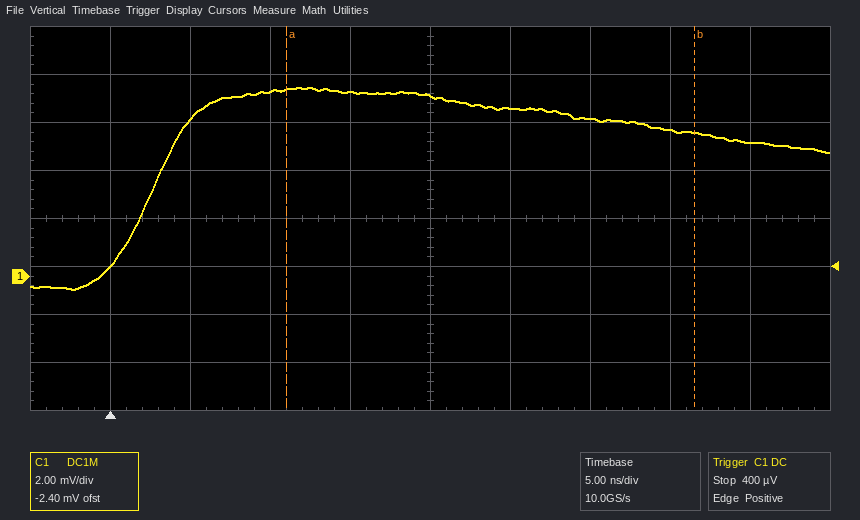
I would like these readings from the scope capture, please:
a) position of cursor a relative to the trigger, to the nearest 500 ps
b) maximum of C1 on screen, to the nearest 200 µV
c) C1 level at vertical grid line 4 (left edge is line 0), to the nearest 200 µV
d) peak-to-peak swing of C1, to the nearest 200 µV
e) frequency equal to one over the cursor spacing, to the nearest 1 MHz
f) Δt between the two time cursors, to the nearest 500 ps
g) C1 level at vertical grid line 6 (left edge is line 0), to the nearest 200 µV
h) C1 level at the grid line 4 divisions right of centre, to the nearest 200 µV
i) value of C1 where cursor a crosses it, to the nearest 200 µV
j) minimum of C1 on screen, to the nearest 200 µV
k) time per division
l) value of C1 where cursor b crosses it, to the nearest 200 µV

+11.0 ns
7.8 mV
7.6 mV
8.4 mV
39 MHz
25.5 ns
7.0 mV
5.6 mV
7.8 mV
-600 µV
5 ns
6.0 mV
